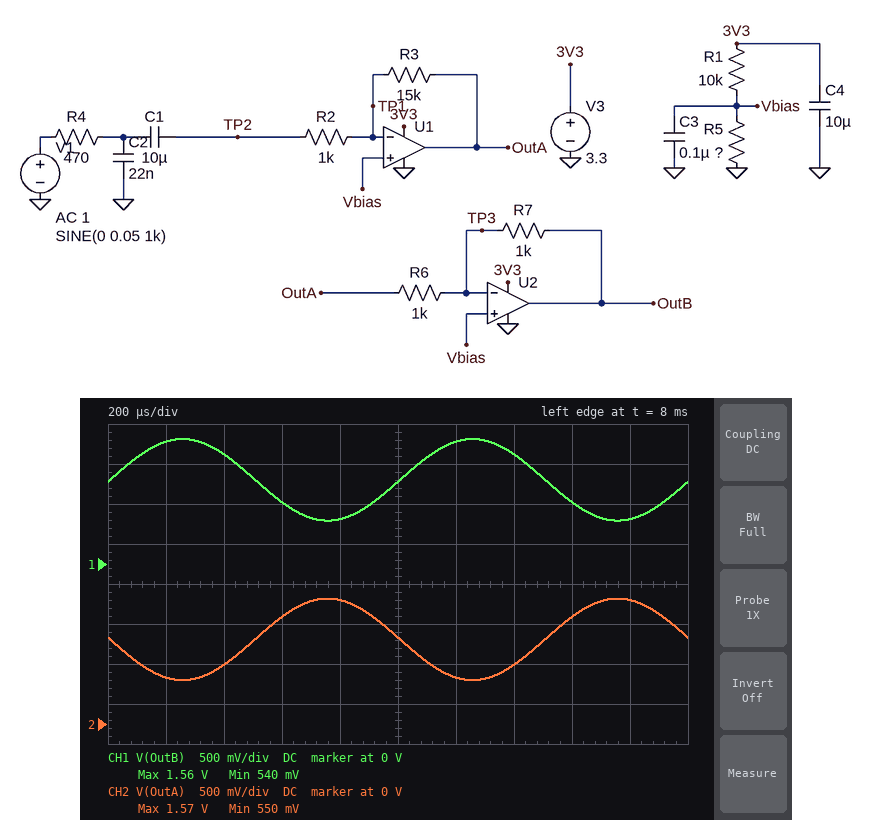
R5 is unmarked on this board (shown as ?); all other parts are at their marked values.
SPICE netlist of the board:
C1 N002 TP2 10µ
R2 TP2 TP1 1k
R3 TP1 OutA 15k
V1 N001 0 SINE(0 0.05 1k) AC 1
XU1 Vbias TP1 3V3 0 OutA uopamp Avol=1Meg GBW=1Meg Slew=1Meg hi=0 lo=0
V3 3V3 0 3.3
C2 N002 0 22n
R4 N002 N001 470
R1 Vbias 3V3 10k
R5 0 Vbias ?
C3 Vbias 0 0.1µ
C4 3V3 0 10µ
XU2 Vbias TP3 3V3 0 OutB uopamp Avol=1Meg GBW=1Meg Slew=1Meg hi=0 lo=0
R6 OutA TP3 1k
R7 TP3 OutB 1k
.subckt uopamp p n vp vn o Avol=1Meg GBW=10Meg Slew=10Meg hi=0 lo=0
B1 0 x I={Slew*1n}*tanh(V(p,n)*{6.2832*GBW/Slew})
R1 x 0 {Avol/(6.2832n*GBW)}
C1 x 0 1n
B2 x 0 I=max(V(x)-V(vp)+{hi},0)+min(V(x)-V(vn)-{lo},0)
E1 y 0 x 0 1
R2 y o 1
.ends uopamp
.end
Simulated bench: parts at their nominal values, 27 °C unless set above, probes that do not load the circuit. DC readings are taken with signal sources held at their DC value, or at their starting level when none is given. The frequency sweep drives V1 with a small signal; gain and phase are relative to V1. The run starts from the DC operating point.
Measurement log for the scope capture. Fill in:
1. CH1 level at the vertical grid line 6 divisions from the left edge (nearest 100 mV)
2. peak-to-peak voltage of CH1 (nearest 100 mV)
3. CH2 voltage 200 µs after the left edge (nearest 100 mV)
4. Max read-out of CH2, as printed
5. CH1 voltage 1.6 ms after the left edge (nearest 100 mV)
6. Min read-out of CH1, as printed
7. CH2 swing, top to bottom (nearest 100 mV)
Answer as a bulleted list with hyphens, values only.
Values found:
- 1.5 V
- 1.0 V
- 600 mV
- 1.57 V
- 800 mV
- 540 mV
- 1.0 V
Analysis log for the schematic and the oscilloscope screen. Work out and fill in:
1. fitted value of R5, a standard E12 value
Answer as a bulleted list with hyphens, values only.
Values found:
- 4.7 kΩ
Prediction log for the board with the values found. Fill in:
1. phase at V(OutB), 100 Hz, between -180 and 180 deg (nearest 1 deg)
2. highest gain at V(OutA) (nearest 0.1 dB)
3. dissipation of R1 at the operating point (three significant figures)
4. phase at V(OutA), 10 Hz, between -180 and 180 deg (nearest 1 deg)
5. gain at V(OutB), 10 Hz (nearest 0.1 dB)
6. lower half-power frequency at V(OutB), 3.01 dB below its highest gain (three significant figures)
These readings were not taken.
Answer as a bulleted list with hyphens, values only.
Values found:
- 6 deg
- 20.2 dB
- 504 µW
- -133 deg
- 16.8 dB
- 10.8 Hz
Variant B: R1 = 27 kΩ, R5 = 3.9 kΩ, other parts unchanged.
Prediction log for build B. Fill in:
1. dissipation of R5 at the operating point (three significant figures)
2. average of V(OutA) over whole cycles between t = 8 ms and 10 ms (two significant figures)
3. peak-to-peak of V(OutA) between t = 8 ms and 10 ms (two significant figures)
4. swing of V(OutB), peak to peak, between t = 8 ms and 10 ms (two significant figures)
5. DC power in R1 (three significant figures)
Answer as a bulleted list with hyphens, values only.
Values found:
- 44.5 µW
- 430 mV
- 920 mV
- 830 mV
- 308 µW
